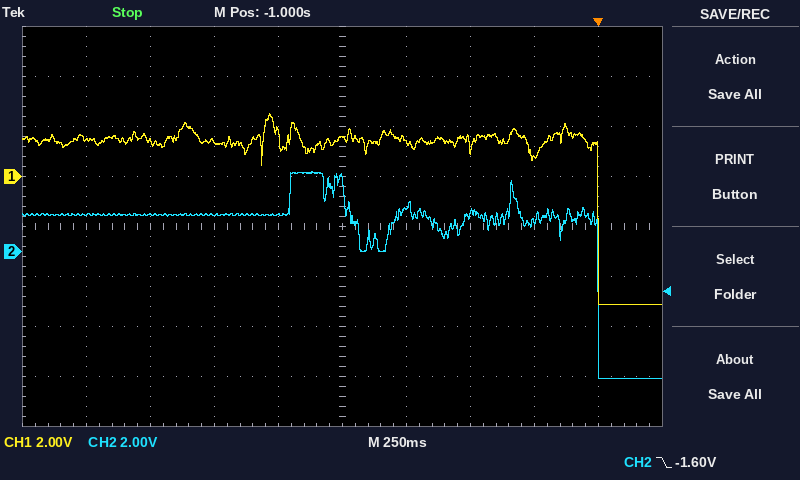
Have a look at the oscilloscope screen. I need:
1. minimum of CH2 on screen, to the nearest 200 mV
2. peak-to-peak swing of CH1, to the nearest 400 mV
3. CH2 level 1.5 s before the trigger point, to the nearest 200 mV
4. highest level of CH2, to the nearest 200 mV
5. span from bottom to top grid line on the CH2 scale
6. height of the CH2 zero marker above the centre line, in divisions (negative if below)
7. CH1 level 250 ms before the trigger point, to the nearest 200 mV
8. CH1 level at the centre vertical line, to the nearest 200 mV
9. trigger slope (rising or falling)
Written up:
-5.0 V
7.6 V
1.4 V
3.2 V
16 V
-0.5 div
800 mV
1.6 V
falling
